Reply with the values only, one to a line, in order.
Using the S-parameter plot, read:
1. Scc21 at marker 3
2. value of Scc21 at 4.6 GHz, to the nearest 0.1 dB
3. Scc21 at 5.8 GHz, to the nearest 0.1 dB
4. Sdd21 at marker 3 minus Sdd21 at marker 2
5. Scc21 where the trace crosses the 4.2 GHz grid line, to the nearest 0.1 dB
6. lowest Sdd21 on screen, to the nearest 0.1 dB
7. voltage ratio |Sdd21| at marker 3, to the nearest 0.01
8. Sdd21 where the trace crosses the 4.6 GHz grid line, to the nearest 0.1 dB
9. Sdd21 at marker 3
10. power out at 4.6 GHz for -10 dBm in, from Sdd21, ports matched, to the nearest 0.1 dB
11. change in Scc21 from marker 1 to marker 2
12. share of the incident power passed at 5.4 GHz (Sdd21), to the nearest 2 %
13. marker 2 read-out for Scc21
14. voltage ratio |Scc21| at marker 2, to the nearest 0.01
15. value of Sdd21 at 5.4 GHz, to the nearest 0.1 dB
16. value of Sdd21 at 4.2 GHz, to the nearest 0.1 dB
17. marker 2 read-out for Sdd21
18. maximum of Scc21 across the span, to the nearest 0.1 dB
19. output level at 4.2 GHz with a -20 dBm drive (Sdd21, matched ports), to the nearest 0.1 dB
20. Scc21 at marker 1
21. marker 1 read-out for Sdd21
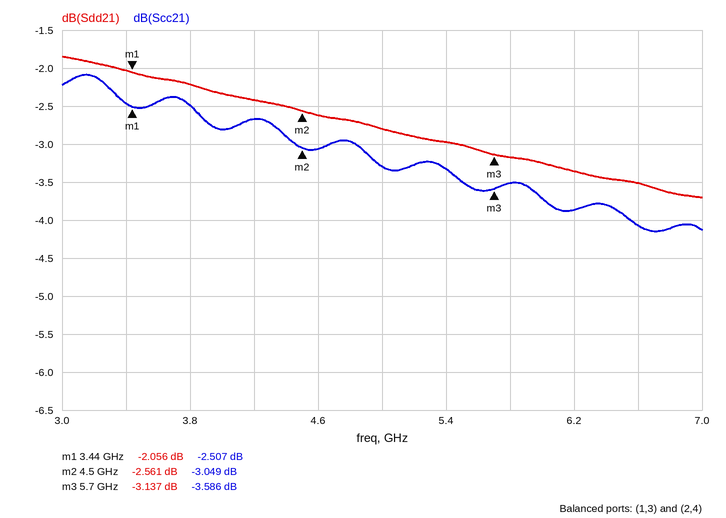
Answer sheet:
-3.586 dB
-3.1 dB
-3.5 dB
-0.576 dB
-2.7 dB
-3.7 dB
0.70
-2.6 dB
-3.137 dB
-12.6 dBm
-0.542 dB
50 %
-3.049 dB
0.70
-3.0 dB
-2.4 dB
-2.561 dB
-2.1 dB
-22.4 dBm
-2.507 dB
-2.056 dB
